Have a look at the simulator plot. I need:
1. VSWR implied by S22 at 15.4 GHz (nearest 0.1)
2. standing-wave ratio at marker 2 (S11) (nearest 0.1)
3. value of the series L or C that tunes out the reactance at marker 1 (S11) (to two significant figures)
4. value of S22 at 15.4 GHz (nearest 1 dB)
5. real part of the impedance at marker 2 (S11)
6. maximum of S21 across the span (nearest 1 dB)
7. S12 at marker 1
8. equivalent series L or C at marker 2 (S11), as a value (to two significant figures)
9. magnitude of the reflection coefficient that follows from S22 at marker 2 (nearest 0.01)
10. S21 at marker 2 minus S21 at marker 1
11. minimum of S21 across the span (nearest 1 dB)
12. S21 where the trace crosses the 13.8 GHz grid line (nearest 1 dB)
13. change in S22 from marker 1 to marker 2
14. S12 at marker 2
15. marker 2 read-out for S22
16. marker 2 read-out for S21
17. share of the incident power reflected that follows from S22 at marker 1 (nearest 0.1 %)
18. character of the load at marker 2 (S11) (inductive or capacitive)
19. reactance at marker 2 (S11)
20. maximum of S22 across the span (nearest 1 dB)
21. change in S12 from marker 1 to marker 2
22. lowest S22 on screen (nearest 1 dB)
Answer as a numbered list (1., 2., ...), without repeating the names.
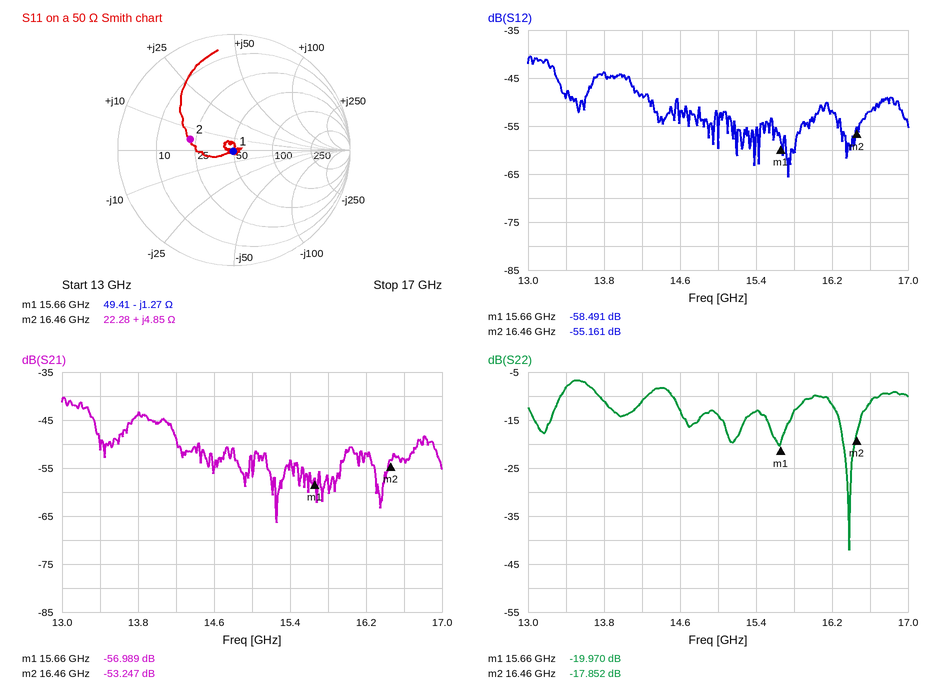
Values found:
1. 1.6
2. 2.3
3. 13 pH
4. -13 dB
5. 22.28 Ω
6. -40 dB
7. -58.491 dB
8. 47 pH
9. 0.13
10. 3.742 dB
11. -66 dB
12. -44 dB
13. 2.118 dB
14. -55.161 dB
15. -17.852 dB
16. -53.247 dB
17. 1.0 %
18. inductive
19. +4.85 Ω
20. -7 dB
21. 3.330 dB
22. -42 dB
